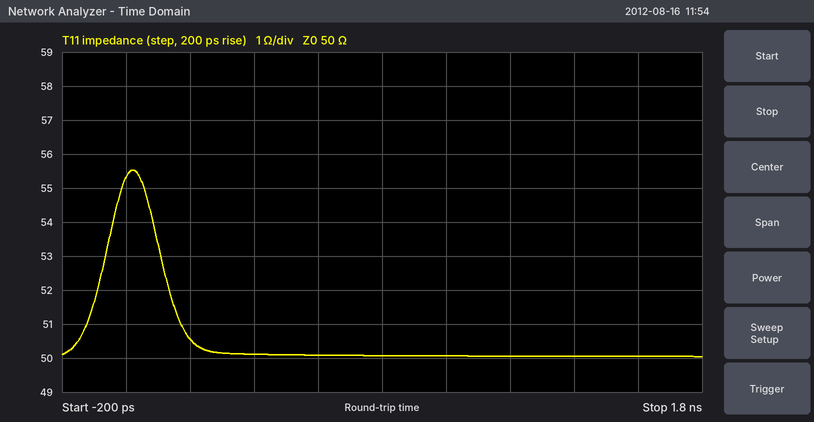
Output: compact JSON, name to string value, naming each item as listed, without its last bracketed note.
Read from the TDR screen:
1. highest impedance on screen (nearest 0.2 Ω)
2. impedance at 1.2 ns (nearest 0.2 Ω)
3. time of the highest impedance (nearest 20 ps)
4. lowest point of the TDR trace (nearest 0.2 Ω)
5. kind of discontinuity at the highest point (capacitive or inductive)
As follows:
{"highest impedance on screen": "55.6 Ω", "impedance at 1.2 ns": "50.0 Ω", "time of the highest impedance": "20 ps", "lowest point of the TDR trace": "50.0 Ω", "kind of discontinuity at the highest point": "inductive"}
